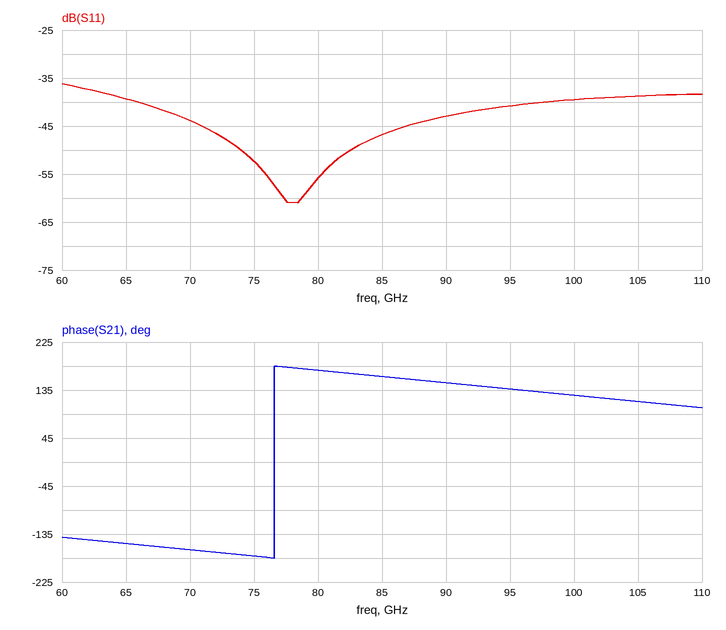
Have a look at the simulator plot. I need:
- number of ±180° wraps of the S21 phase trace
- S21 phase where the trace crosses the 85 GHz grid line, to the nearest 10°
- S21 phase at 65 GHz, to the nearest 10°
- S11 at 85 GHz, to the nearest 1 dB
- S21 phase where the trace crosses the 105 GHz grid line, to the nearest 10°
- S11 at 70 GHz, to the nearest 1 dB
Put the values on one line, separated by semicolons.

1; 160°; -150°; -47 dB; 110°; -44 dB
